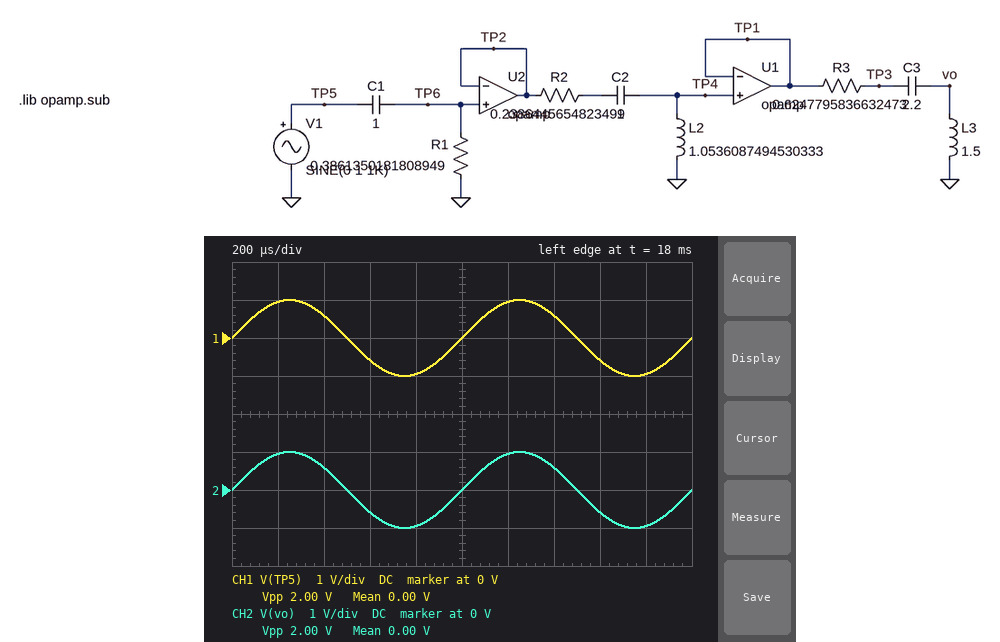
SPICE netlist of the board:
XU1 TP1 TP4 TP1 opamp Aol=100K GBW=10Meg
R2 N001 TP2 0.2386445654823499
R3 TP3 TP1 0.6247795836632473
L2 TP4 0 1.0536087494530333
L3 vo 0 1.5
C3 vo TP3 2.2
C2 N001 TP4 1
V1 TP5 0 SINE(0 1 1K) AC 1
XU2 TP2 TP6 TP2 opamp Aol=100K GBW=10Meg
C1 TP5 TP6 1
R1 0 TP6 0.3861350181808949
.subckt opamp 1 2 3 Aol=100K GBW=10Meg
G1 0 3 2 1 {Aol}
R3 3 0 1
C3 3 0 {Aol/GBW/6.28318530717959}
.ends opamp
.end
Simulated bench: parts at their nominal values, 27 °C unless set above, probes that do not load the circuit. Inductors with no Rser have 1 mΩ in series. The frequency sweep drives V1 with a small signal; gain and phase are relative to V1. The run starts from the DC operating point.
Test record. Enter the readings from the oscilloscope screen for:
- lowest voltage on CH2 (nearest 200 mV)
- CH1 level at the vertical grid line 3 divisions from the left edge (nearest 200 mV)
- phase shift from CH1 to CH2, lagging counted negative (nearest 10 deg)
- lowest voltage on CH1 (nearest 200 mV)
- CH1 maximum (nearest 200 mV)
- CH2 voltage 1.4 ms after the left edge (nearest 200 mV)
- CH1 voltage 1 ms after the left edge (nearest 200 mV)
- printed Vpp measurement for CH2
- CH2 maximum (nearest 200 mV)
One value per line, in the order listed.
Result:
-1.0 V
-600 mV
0 deg
-1.0 V
1.0 V
600 mV
0 V
2.00 V
1.0 V
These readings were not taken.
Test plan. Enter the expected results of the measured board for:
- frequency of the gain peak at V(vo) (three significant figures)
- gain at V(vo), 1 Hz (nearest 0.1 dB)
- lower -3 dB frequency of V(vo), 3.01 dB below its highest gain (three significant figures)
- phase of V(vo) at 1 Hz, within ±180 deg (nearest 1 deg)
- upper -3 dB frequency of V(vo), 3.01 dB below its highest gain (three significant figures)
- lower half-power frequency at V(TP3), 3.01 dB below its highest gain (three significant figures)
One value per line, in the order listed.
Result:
158 mHz
-0.4 dB
143 mHz
28 deg
185 mHz
145 mHz
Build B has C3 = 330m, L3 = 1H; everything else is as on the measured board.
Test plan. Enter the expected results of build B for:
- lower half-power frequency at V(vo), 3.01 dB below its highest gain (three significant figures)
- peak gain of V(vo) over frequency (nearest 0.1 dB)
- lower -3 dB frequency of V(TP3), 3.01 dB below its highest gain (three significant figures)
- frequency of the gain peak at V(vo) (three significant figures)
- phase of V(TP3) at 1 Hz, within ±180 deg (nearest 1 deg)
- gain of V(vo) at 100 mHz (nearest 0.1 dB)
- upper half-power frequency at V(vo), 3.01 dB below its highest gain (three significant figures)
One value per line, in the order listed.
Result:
241 mHz
7.0 dB
143 mHz
285 mHz
31 deg
-32.4 dB
366 mHz
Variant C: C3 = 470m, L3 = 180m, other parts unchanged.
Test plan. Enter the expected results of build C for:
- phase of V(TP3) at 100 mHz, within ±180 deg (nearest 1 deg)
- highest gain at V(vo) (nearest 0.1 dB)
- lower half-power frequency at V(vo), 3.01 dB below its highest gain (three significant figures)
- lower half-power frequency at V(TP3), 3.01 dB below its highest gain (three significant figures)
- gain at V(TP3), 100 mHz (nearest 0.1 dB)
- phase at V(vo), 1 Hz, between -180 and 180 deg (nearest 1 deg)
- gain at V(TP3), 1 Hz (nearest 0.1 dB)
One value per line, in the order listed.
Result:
-129 deg
0.5 dB
498 mHz
143 mHz
-15.9 dB
63 deg
-2.6 dB
